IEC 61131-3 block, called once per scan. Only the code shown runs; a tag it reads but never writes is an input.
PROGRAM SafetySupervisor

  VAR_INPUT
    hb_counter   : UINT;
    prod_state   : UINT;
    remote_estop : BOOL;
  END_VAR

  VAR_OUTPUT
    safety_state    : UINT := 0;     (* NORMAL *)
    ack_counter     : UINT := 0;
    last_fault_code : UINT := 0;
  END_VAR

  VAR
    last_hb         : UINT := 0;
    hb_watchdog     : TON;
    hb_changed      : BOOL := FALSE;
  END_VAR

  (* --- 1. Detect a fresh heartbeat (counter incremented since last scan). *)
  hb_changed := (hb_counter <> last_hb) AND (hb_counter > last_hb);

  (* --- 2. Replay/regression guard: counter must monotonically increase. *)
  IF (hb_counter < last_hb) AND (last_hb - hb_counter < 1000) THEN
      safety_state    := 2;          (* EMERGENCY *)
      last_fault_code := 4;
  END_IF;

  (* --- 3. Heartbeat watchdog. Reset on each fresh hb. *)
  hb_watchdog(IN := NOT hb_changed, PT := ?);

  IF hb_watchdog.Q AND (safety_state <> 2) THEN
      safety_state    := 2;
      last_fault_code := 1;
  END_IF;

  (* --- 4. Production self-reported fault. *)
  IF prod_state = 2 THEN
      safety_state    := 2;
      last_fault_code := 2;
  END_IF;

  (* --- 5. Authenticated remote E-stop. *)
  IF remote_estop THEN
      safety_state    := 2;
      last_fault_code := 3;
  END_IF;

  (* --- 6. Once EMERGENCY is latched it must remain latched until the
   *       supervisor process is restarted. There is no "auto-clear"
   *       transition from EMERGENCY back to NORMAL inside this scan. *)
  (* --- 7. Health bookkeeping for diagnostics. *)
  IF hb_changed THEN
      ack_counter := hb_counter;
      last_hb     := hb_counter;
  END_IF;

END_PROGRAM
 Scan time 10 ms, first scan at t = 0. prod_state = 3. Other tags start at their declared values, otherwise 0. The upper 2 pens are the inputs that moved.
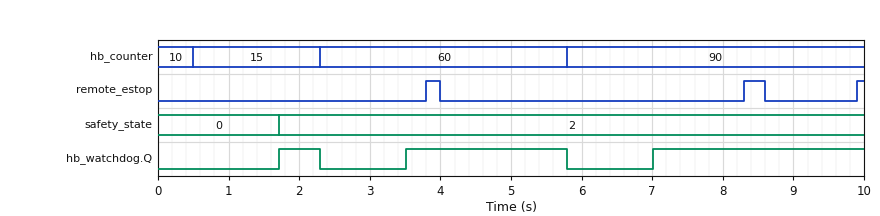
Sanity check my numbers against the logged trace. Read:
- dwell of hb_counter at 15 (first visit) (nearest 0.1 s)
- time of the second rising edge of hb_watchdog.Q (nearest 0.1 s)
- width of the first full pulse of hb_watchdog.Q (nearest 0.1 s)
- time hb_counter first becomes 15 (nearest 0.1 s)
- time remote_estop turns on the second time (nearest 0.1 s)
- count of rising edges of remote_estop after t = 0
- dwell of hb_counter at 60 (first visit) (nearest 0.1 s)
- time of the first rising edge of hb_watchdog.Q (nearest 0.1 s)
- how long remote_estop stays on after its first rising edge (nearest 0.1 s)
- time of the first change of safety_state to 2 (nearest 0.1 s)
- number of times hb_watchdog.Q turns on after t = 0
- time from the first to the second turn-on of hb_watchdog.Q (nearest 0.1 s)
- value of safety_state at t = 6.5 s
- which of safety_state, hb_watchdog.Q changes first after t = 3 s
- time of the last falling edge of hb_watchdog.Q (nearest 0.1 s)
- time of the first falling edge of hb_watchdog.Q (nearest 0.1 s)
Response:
1.8 s
3.5 s
0.6 s
0.5 s
8.3 s
3
3.5 s
1.7 s
0.2 s
1.7 s
3
1.8 s
2
hb_watchdog.Q
5.8 s
2.3 s
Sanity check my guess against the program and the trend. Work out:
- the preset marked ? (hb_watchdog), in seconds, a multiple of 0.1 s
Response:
1.2 s
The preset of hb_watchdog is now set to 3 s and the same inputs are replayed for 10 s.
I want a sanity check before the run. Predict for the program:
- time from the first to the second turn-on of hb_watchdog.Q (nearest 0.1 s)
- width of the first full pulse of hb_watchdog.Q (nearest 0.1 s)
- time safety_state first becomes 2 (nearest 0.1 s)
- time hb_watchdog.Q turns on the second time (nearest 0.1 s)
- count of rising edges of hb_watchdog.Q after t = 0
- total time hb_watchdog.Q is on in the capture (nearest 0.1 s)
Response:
3.5 s
0.5 s
3.8 s
8.8 s
2
1.7 s
